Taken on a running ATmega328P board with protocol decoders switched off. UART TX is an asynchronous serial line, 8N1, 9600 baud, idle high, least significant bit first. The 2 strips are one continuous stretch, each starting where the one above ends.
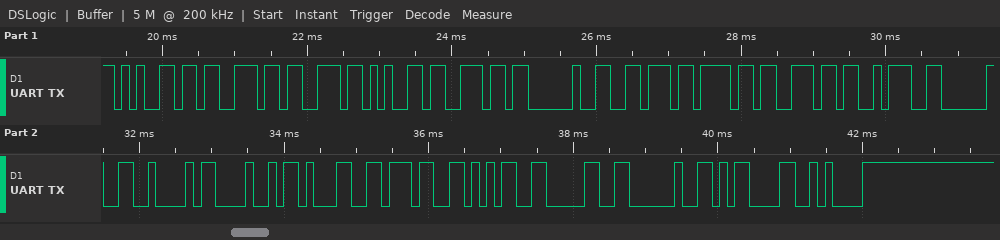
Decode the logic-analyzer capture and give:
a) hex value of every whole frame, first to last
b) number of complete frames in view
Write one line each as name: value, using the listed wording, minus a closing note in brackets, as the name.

hex value of every whole frame, first to last: 65 73 73 65 6E 20 76 6F 6E 3A 20 42 48 31 37 35 30 20 0D 0A
number of complete frames in view: 20
